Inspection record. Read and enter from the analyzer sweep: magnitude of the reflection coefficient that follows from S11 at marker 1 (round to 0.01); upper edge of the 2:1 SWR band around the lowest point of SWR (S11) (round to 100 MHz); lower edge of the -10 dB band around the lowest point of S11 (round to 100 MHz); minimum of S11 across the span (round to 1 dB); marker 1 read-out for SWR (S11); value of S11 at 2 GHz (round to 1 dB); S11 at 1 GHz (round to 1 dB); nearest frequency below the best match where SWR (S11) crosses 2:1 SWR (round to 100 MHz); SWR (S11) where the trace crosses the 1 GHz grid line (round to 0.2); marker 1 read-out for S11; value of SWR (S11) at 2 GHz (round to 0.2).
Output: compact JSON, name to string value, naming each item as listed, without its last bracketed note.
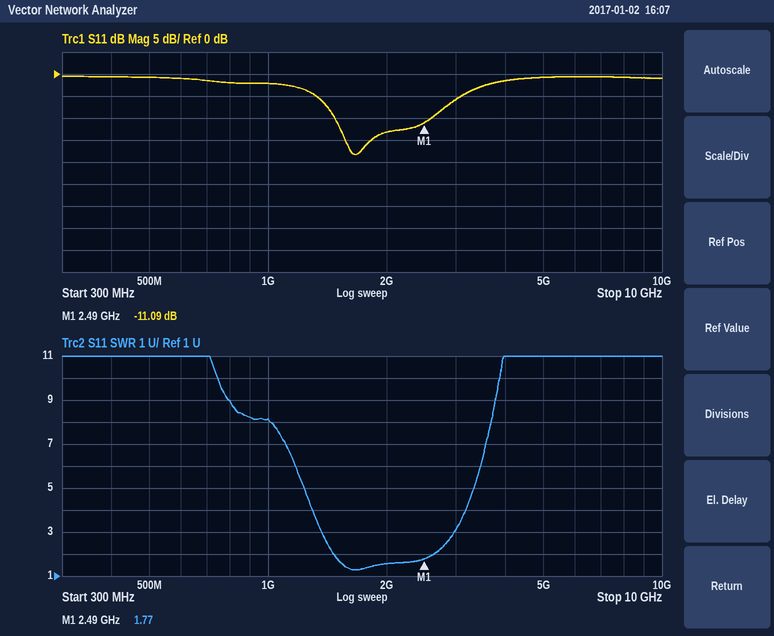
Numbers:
{"magnitude of the reflection coefficient that follows from S11 at marker 1": "0.28", "upper edge of the 2:1 SWR band around the lowest point of SWR (S11)": "2.6 GHz", "lower edge of the -10 dB band around the lowest point of S11": "1.5 GHz", "minimum of S11 across the span": "-18 dB", "marker 1 read-out for SWR": "1.77", "value of S11 at 2 GHz": "-13 dB", "S11 at 1 GHz": "-2 dB", "nearest frequency below the best match where SWR (S11) crosses 2:1 SWR": "1.5 GHz", "SWR (S11) where the trace crosses the 1 GHz grid line": "8.2", "marker 1 read-out for S11": "-11.09 dB", "value of SWR (S11) at 2 GHz": "1.6"}
